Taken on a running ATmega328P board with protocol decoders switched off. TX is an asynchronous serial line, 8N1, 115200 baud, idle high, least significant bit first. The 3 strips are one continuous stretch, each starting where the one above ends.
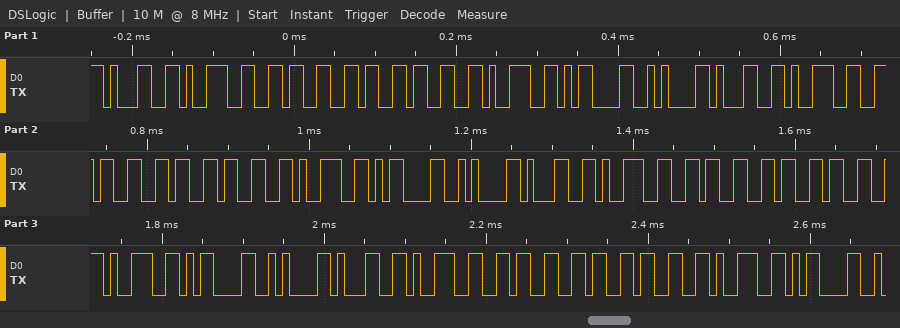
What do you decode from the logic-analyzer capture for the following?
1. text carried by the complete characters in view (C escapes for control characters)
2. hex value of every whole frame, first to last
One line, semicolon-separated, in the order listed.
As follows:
"196639\r\n196639\r\n196639\r\n196639\r"; 31 39 36 36 33 39 0D 0A 31 39 36 36 33 39 0D 0A 31 39 36 36 33 39 0D 0A 31 39 36 36 33 39 0D
